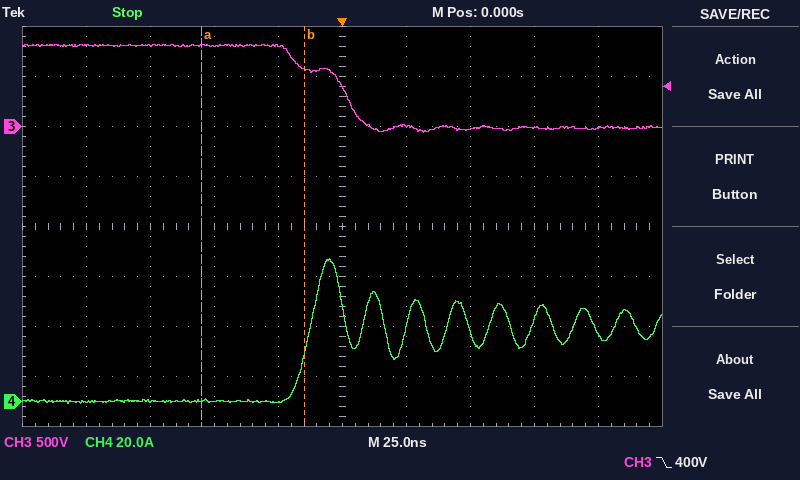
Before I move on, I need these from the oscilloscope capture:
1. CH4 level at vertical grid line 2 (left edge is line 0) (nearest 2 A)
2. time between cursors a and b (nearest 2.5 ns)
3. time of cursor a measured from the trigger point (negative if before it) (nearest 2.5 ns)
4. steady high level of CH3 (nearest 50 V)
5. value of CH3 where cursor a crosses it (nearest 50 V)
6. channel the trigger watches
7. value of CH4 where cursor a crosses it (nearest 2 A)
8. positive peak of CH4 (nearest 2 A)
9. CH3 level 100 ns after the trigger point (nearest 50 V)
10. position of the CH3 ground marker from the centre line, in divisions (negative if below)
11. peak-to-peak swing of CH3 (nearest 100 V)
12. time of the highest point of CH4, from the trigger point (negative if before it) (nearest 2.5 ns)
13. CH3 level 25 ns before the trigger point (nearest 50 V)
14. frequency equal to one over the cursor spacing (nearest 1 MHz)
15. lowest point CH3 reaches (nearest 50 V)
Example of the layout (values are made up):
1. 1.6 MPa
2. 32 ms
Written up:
1. 0 A
2. 40.0 ns
3. -55.0 ns
4. 800 V
5. 800 V
6. CH3
7. 0 A
8. 58 A
9. 0 V
10. +2.0 div
11. 900 V
12. -5.0 ns
13. 800 V
14. 25 MHz
15. -50 V
